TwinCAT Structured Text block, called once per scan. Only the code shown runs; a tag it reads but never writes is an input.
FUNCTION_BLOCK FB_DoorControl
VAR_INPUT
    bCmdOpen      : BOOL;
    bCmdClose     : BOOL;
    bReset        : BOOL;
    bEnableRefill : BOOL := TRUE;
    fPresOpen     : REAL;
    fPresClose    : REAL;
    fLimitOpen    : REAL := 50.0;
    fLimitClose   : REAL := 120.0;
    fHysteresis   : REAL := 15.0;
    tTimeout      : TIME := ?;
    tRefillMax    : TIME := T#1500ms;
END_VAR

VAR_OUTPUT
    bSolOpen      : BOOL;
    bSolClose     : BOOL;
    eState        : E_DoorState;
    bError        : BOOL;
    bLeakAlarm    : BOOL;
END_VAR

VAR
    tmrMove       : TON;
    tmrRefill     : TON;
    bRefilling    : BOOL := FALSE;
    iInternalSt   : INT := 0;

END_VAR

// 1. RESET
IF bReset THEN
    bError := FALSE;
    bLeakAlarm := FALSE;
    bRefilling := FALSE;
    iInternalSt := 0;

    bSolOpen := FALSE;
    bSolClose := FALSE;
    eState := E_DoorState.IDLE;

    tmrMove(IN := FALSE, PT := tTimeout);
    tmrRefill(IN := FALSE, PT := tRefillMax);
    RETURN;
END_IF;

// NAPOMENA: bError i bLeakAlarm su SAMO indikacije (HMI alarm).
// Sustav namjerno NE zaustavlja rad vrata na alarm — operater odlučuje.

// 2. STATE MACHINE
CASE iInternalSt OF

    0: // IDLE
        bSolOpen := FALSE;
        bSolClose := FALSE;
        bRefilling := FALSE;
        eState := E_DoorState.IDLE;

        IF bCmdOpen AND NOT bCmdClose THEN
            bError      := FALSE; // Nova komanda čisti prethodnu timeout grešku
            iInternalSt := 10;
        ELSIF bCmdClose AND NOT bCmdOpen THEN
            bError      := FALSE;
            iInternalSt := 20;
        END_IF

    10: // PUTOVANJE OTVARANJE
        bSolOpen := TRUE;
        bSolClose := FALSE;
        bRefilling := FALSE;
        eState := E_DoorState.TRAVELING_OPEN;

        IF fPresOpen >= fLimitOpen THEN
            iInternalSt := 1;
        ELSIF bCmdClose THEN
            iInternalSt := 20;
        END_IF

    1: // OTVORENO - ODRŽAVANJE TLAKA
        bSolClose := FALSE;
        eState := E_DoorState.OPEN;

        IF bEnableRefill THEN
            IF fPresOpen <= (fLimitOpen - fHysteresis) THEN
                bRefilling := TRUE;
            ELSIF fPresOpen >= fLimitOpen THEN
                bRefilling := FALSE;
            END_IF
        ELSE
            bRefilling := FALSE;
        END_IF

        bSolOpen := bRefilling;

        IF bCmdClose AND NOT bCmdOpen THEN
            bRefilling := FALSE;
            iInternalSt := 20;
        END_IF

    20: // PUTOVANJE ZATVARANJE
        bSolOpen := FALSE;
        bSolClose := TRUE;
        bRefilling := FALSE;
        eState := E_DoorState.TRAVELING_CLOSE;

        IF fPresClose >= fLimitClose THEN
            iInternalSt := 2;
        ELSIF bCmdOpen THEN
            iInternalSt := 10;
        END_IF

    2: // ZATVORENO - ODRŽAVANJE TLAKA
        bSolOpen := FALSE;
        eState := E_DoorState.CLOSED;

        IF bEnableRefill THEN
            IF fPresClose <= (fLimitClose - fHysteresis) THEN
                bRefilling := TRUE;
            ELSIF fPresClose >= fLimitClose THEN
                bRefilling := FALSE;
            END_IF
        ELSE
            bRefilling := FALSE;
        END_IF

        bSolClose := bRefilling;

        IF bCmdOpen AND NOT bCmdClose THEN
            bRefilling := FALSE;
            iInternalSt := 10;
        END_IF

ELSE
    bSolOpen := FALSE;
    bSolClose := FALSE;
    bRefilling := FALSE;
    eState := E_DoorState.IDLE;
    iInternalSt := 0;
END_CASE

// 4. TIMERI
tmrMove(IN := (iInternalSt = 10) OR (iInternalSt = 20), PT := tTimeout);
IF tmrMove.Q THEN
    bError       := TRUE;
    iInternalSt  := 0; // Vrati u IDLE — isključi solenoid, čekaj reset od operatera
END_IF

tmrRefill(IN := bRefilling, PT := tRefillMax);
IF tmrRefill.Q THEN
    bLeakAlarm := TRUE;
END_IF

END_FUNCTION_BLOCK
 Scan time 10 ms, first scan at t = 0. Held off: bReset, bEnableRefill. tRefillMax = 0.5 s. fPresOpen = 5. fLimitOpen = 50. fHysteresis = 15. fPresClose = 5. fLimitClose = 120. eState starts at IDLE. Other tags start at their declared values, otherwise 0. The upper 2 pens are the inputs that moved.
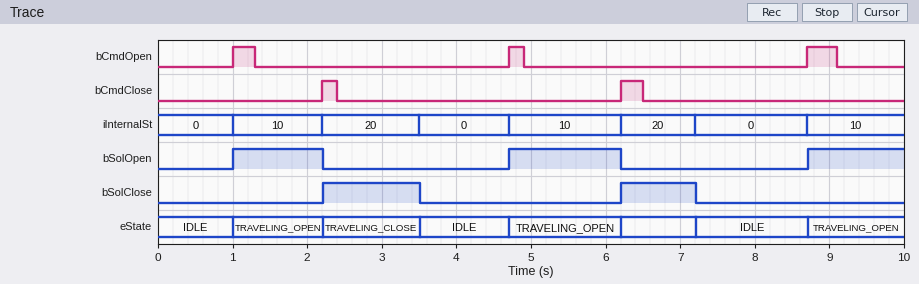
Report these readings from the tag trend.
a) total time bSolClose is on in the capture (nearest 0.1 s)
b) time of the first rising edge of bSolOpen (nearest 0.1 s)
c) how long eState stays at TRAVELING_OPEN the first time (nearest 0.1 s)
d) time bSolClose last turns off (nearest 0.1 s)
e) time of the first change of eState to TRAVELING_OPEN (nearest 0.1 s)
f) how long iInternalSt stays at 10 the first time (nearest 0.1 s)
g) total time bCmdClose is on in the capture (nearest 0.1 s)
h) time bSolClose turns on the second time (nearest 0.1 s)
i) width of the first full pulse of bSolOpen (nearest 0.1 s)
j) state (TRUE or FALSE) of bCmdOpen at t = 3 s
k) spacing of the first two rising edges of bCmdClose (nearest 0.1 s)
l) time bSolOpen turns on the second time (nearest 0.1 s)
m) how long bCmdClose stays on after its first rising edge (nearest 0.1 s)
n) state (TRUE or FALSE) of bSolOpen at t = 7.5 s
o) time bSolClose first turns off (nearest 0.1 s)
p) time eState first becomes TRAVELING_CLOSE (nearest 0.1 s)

2.3 s
1.0 s
1.2 s
7.2 s
1.0 s
1.2 s
0.5 s
6.2 s
1.2 s
FALSE
4.0 s
4.7 s
0.2 s
FALSE
3.5 s
2.2 s
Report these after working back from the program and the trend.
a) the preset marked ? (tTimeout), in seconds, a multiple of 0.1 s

2.5 s
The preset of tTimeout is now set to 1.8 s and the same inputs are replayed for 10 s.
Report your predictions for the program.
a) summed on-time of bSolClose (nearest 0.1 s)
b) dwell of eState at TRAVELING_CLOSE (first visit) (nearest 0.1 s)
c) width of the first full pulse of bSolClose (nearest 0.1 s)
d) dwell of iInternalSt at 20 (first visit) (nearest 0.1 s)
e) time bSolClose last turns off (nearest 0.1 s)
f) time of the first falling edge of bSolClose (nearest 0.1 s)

0.9 s
0.6 s
0.6 s
0.6 s
6.5 s
2.8 s
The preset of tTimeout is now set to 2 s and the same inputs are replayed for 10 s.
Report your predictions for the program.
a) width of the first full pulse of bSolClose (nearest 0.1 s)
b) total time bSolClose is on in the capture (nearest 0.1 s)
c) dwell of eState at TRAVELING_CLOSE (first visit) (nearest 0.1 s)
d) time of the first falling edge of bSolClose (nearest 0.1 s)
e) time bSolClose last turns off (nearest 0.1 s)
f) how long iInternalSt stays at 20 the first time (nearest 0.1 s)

0.8 s
1.3 s
0.8 s
3.0 s
6.7 s
0.8 s
